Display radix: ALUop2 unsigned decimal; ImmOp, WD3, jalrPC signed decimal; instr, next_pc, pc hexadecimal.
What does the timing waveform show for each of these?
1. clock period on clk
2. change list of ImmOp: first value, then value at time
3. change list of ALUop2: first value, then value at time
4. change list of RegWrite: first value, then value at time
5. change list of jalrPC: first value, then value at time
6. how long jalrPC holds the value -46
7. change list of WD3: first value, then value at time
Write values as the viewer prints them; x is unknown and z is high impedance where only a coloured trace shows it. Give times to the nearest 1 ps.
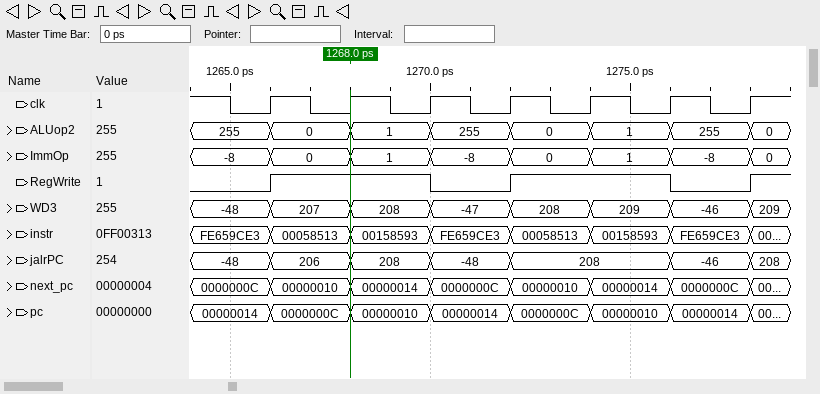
2 ps
-8, 0 at 1266 ps, 1 at 1268 ps, -8 at 1270 ps, 0 at 1272 ps, 1 at 1274 ps, -8 at 1276 ps, 0 at 1278 ps
255, 0 at 1266 ps, 1 at 1268 ps, 255 at 1270 ps, 0 at 1272 ps, 1 at 1274 ps, 255 at 1276 ps, 0 at 1278 ps
0, 1 at 1266 ps, 0 at 1270 ps, 1 at 1272 ps, 0 at 1276 ps, 1 at 1278 ps
-48, 206 at 1266 ps, 208 at 1268 ps, -48 at 1270 ps, 208 at 1272 ps, -46 at 1276 ps, 208 at 1278 ps
2 ps
-48, 207 at 1266 ps, 208 at 1268 ps, -47 at 1270 ps, 208 at 1272 ps, 209 at 1274 ps, -46 at 1276 ps, 209 at 1278 ps
